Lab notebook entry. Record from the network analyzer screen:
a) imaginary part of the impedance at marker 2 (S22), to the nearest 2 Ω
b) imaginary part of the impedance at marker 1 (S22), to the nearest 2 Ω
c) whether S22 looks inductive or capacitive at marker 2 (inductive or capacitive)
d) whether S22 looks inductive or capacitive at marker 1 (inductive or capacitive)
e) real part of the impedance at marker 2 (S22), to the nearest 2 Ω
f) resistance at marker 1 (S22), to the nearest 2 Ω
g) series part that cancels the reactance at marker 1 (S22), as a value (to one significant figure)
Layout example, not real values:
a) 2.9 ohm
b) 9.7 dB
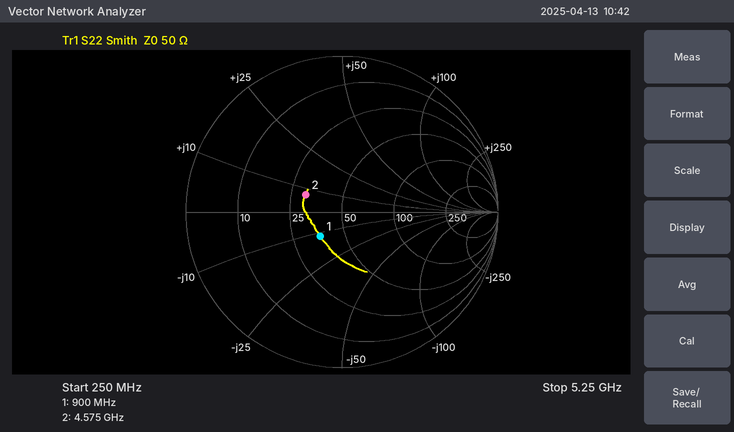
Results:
a) +8 Ω
b) -12 Ω
c) inductive
d) capacitive
e) 30 Ω
f) 36 Ω
g) 2 nH
